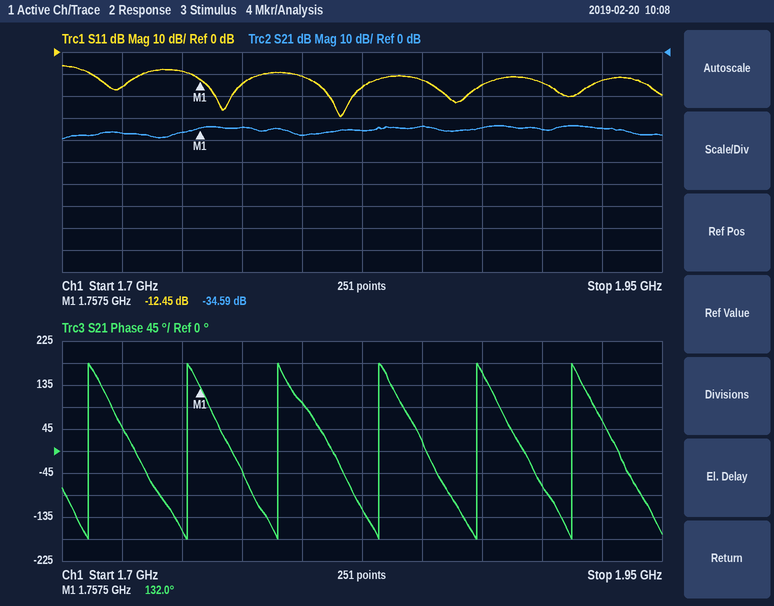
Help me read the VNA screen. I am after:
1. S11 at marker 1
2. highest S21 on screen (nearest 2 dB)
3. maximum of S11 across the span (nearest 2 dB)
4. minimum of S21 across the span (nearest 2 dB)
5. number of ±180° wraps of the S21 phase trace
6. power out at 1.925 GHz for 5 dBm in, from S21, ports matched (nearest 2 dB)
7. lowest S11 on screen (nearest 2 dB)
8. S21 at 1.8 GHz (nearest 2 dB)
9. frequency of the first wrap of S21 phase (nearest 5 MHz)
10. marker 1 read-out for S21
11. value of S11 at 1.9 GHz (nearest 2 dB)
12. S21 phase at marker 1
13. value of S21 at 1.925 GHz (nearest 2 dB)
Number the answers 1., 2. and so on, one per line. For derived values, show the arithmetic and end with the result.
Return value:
1. -12.45 dB
2. -34 dB
3. -6 dB
4. -40 dB
5. 6
6. 5 dBm + (-34 dB) = -30 dBm
7. -30 dB
8. -38 dB
9. 1.710 GHz
10. -34.59 dB
11. -14 dB
12. 132.0°
13. -34 dB
